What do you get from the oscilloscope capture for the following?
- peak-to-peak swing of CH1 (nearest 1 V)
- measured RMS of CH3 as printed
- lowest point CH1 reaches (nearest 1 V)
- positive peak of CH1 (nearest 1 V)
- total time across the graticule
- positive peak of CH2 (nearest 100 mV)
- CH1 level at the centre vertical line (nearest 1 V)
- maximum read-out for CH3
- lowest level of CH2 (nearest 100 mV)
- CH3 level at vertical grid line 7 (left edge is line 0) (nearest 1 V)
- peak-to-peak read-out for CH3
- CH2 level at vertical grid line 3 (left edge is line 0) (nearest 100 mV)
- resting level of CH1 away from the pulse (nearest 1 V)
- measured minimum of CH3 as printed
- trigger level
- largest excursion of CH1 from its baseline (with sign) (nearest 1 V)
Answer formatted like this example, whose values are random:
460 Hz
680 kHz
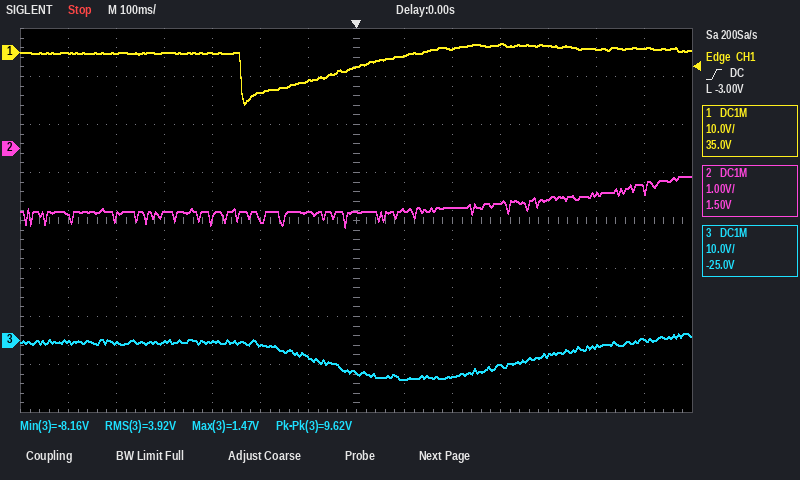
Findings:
13 V
3.92 V
-11 V
2 V
1.4 s
-600 mV
-3 V
1.47 V
-1.6 V
-7 V
9.62 V
-1.3 V
0 V
-8.16 V
-3.00 V
-11 V
